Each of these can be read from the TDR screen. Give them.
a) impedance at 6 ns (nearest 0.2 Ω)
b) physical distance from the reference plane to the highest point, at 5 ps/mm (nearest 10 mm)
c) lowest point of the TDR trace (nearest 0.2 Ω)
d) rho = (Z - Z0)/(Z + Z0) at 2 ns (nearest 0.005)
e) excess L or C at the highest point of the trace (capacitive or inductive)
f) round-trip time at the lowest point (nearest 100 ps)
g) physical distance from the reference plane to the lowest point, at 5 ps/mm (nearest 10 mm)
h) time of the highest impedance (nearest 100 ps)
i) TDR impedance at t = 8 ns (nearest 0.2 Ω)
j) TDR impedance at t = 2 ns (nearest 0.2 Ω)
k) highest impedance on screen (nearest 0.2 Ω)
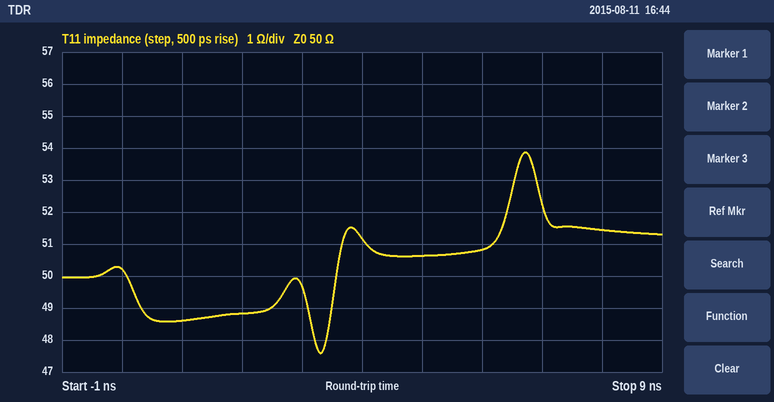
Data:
50.8 Ω
670 mm
47.6 Ω
-0.010
inductive
3.3 ns
330 mm
6.7 ns
51.4 Ω
48.8 Ω
53.8 Ω
